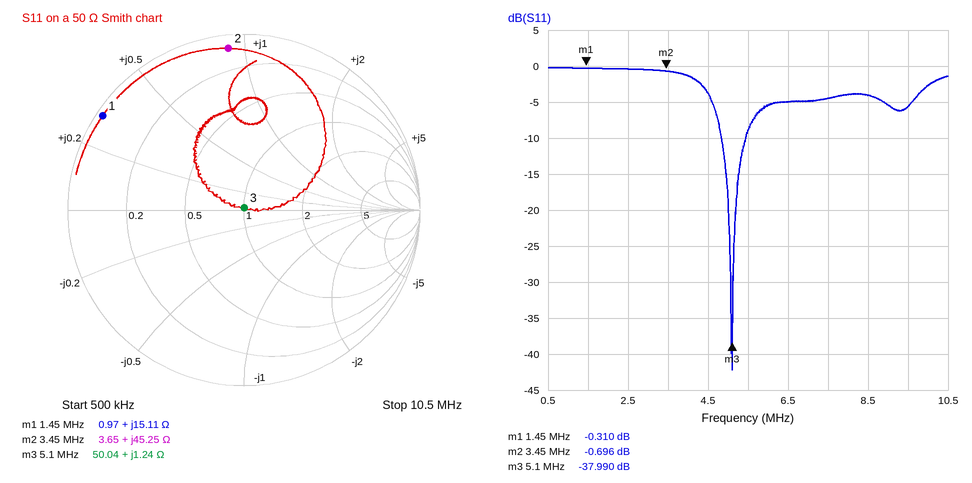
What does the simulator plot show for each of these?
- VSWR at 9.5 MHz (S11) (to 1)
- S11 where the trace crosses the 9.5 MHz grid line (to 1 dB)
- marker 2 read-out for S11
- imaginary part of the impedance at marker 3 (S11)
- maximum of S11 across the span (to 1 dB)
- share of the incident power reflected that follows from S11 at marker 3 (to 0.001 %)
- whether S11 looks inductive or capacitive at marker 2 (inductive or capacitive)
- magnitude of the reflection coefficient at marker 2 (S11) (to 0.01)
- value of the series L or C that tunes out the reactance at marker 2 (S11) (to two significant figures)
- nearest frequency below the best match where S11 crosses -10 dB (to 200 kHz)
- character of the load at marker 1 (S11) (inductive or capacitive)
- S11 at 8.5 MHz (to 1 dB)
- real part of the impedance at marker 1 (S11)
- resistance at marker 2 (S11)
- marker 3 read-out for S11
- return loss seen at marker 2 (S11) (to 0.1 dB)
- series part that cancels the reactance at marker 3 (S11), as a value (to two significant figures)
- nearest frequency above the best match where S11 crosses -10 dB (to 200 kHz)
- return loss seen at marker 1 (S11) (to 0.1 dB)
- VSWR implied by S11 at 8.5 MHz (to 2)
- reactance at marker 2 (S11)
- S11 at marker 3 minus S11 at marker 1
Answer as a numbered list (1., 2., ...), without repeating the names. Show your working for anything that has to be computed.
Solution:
1. |Γ| = 10^(-6/20) = 0.5012; VSWR = (1 + 0.5012)/(1 − 0.5012) ≈ 3
2. -6 dB
3. -0.696 dB
4. +1.24 Ω
5. 0 dB
6. 10^(-37.99/10) ≈ 0.016 %
7. inductive
8. 10^(-0.696/20) ≈ 0.92
9. C = 1/(2π × 3.45 MHz × 45.25 Ω) ≈ 1.0 nF
10. 4.8 MHz
11. inductive
12. -4 dB
13. 0.97 Ω
14. 3.65 Ω
15. -37.990 dB
16. 0.7 dB
17. C = 1/(2π × 5.1 MHz × 1.24 Ω) ≈ 25 nF
18. 5.4 MHz
19. 0.3 dB
20. |Γ| = 10^(-4/20) = 0.6310; VSWR = (1 + 0.6310)/(1 − 0.6310) ≈ 4
21. +45.25 Ω
22. -37.99 − (-0.31) = -37.680 dB
